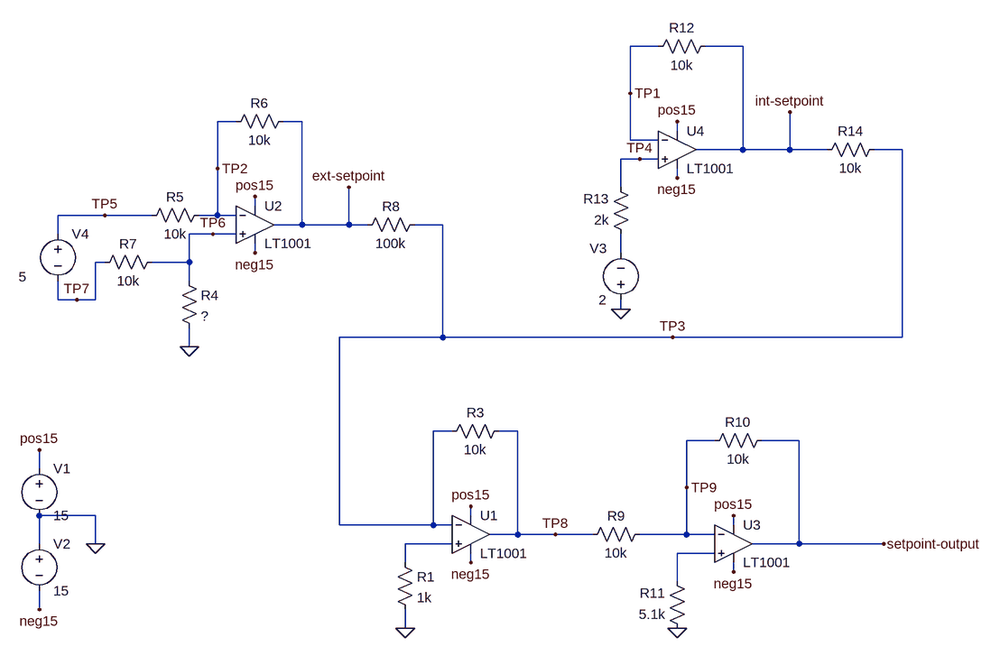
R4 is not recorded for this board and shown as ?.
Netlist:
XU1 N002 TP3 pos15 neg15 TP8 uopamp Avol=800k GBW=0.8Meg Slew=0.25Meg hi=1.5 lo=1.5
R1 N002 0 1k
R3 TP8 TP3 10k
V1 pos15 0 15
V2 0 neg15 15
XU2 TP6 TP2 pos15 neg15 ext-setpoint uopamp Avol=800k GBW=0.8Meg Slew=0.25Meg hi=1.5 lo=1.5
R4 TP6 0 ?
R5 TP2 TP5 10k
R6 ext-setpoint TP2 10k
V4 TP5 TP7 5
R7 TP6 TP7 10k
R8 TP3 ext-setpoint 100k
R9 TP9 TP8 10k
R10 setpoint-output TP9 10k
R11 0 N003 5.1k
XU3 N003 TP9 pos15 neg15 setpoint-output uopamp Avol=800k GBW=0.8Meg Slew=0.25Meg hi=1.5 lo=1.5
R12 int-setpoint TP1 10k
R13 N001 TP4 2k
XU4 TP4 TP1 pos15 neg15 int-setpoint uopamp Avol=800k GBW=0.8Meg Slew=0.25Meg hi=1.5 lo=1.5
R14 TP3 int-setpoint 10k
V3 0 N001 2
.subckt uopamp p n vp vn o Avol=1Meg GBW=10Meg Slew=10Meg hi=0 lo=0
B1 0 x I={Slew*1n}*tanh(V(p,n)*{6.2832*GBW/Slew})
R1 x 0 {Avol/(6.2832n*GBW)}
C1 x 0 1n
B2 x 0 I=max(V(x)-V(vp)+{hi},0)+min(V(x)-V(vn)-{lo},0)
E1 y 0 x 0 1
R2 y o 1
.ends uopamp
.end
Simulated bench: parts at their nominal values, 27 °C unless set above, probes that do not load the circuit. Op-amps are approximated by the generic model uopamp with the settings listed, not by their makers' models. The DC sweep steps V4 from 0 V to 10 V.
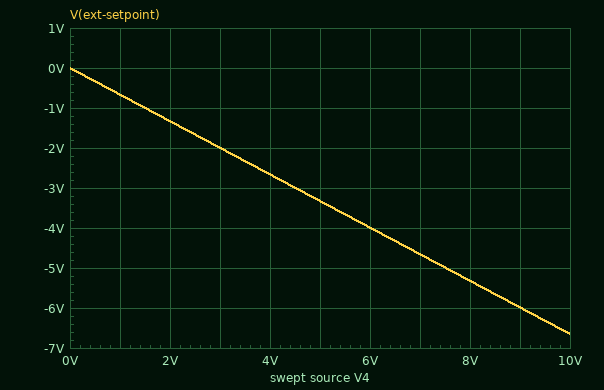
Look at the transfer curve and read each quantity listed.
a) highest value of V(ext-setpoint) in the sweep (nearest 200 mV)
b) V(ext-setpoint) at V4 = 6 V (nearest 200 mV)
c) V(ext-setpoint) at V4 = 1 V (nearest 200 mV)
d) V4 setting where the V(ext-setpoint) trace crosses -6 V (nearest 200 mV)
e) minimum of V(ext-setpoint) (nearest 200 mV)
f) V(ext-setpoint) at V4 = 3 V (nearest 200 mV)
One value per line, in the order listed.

0 V
-4.0 V
-600 mV
9.0 V
-6.6 V
-2.0 V
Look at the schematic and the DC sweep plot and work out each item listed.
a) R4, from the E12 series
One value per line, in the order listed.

3.3 kΩ
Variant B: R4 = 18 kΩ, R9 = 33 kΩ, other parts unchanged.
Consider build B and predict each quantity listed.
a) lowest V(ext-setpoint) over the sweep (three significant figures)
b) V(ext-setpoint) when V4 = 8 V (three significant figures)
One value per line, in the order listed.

-13.5 V
-11.2 V
